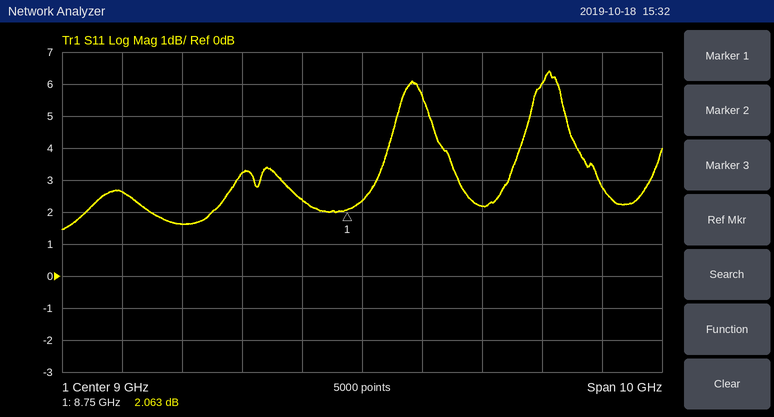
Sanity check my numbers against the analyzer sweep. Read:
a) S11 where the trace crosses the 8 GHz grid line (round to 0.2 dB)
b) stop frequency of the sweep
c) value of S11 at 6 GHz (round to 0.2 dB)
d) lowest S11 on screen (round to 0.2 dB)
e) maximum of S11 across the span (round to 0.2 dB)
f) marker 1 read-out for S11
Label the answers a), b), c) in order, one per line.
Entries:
a) 2.4 dB
b) 14 GHz
c) 1.6 dB
d) 1.4 dB
e) 6.4 dB
f) 2.063 dB
